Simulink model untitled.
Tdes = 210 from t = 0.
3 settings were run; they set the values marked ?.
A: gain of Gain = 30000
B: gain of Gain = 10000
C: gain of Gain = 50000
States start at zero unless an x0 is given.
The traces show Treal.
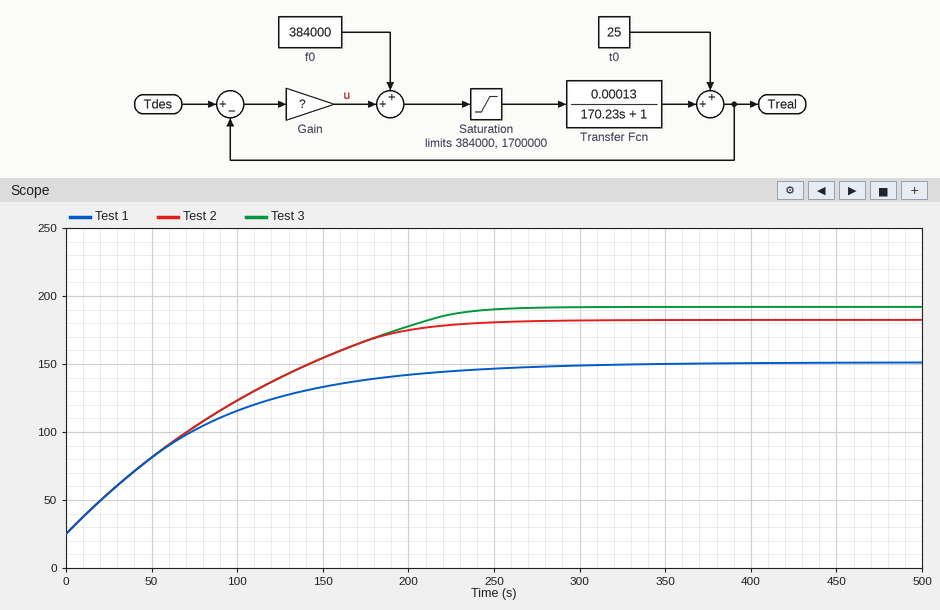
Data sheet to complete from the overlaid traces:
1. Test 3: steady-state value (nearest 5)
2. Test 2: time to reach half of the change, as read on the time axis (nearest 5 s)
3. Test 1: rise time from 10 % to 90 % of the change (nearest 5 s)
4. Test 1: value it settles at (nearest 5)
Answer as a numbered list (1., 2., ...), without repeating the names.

1. 190
2. 75 s
3. 165 s
4. 150
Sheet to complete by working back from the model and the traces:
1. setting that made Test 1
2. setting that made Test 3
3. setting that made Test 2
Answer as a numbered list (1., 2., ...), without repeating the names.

1. B
2. C
3. A
